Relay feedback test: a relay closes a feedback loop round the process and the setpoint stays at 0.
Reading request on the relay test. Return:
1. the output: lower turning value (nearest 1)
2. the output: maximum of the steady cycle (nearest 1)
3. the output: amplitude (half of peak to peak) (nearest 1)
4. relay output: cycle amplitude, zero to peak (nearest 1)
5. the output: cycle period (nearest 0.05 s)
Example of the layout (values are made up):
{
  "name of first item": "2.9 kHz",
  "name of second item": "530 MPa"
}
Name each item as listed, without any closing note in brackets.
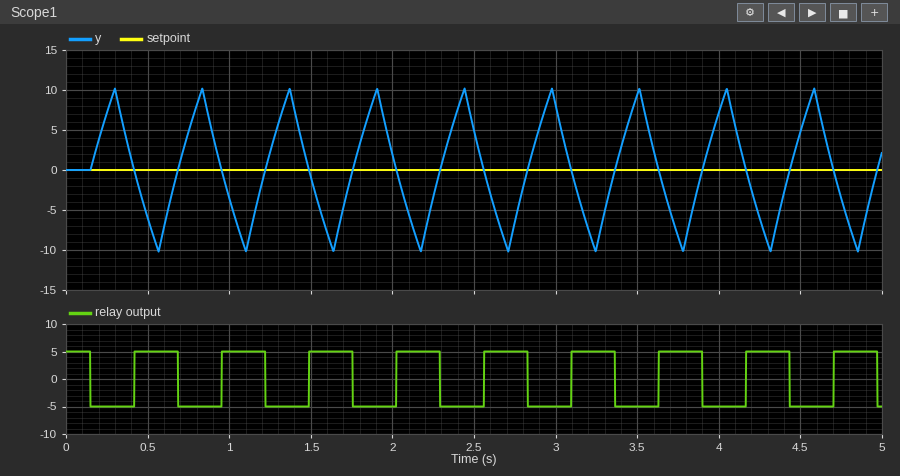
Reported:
{
  "the output: lower turning value": "-10",
  "the output: maximum of the steady cycle": "10",
  "the output: amplitude (half of peak to peak)": "10",
  "relay output: cycle amplitude, zero to peak": "5",
  "the output: cycle period": "0.55 s"
}
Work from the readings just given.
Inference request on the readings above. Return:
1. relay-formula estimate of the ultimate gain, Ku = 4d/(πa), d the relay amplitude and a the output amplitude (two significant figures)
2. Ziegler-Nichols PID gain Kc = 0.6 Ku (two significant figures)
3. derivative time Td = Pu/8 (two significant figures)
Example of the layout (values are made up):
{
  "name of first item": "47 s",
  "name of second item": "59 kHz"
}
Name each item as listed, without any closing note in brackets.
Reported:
{
  "relay-formula estimate of the ultimate gain, Ku = 4d/(πa), d the relay amplitude and a the output amplitude": "0.64",
  "Ziegler-Nichols PID gain Kc = 0.6 Ku": "0.38",
  "derivative time Td = Pu/8": "0.069 s"
}
